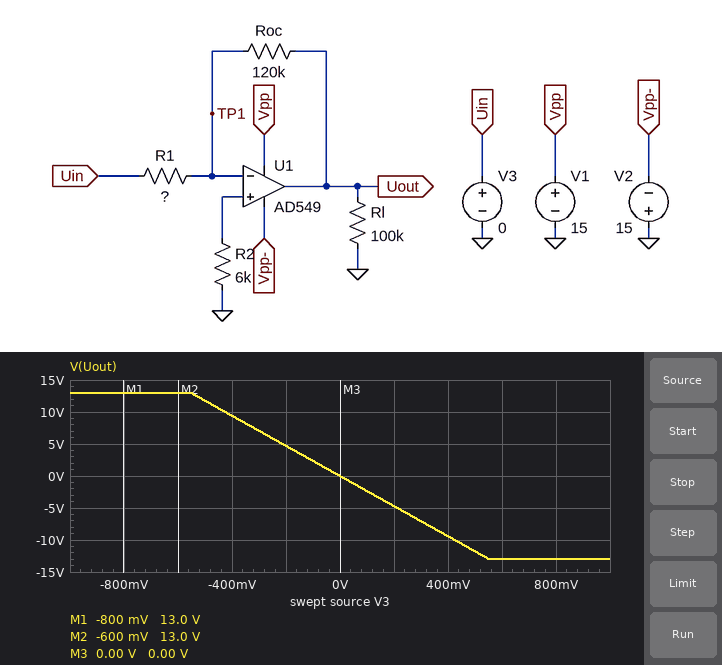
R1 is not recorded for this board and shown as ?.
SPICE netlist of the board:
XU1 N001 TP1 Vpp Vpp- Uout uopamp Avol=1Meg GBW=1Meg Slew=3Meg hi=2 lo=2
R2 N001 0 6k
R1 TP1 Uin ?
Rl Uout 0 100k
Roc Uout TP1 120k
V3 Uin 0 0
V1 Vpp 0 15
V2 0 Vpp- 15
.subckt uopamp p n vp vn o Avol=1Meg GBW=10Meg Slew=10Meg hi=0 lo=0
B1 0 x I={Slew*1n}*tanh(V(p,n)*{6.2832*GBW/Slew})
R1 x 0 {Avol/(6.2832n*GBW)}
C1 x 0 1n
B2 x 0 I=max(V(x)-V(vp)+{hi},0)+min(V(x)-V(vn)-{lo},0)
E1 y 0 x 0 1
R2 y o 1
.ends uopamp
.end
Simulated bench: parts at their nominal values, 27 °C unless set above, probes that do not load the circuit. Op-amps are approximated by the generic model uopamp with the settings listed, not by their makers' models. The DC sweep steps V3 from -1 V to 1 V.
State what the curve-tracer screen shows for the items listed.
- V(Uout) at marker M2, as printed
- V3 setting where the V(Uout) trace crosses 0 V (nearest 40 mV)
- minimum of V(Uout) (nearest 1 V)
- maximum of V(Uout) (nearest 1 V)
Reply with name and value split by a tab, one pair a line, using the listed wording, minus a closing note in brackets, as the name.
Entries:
V(Uout) at marker M2, as printed	13.0 V
V3 setting where the V(Uout) trace crosses 0 V	0 V
minimum of V(Uout)	-13 V
maximum of V(Uout)	13 V
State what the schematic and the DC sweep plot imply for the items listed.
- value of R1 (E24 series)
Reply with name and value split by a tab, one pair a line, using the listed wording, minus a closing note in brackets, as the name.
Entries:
value of R1	5.1 kΩ
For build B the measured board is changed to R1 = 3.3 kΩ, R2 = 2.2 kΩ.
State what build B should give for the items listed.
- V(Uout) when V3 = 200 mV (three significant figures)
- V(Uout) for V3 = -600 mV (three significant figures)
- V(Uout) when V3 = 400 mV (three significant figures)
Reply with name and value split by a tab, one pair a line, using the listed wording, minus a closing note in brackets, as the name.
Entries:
V(Uout) when V3 = 200 mV	-7.27 V
V(Uout) for V3 = -600 mV	13.0 V
V(Uout) when V3 = 400 mV	-13.0 V
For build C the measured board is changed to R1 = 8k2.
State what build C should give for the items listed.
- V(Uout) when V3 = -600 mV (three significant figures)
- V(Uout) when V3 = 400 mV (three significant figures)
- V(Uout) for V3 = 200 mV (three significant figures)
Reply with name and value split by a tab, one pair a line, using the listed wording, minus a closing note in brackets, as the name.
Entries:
V(Uout) when V3 = -600 mV	8.78 V
V(Uout) when V3 = 400 mV	-5.85 V
V(Uout) for V3 = 200 mV	-2.93 V
